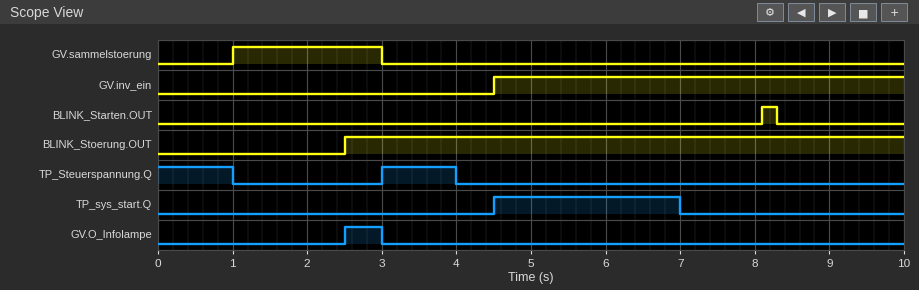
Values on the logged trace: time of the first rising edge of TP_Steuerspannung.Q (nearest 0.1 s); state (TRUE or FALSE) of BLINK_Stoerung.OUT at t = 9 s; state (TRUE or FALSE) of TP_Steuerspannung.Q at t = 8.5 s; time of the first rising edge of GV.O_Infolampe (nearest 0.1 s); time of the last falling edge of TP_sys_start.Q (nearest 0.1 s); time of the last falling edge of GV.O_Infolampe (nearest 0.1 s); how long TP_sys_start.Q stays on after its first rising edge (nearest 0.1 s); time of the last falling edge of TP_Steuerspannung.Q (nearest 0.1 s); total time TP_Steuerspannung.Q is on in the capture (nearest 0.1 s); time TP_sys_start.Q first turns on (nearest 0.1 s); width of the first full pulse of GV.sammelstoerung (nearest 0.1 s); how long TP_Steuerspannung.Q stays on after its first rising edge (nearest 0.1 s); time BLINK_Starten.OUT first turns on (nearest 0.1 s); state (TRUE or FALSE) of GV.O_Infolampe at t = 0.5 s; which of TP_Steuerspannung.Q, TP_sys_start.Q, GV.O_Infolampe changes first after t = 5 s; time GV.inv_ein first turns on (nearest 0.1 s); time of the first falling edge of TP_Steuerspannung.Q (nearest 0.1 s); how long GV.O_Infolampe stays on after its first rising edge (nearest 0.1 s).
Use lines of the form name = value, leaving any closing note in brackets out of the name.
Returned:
time of the first rising edge of TP_Steuerspannung.Q = 3.0 s
state (TRUE or FALSE) of BLINK_Stoerung.OUT at t = 9 s = TRUE
state (TRUE or FALSE) of TP_Steuerspannung.Q at t = 8.5 s = FALSE
time of the first rising edge of GV.O_Infolampe = 2.5 s
time of the last falling edge of TP_sys_start.Q = 7.0 s
time of the last falling edge of GV.O_Infolampe = 3.0 s
how long TP_sys_start.Q stays on after its first rising edge = 2.5 s
time of the last falling edge of TP_Steuerspannung.Q = 4.0 s
total time TP_Steuerspannung.Q is on in the capture = 2.0 s
time TP_sys_start.Q first turns on = 4.5 s
width of the first full pulse of GV.sammelstoerung = 2.0 s
how long TP_Steuerspannung.Q stays on after its first rising edge = 1.0 s
time BLINK_Starten.OUT first turns on = 8.1 s
state (TRUE or FALSE) of GV.O_Infolampe at t = 0.5 s = FALSE
which of TP_Steuerspannung.Q, TP_sys_start.Q, GV.O_Infolampe changes first after t = 5 s = TP_sys_start.Q
time GV.inv_ein first turns on = 4.5 s
time of the first falling edge of TP_Steuerspannung.Q = 1.0 s
how long GV.O_Infolampe stays on after its first rising edge = 0.5 s
